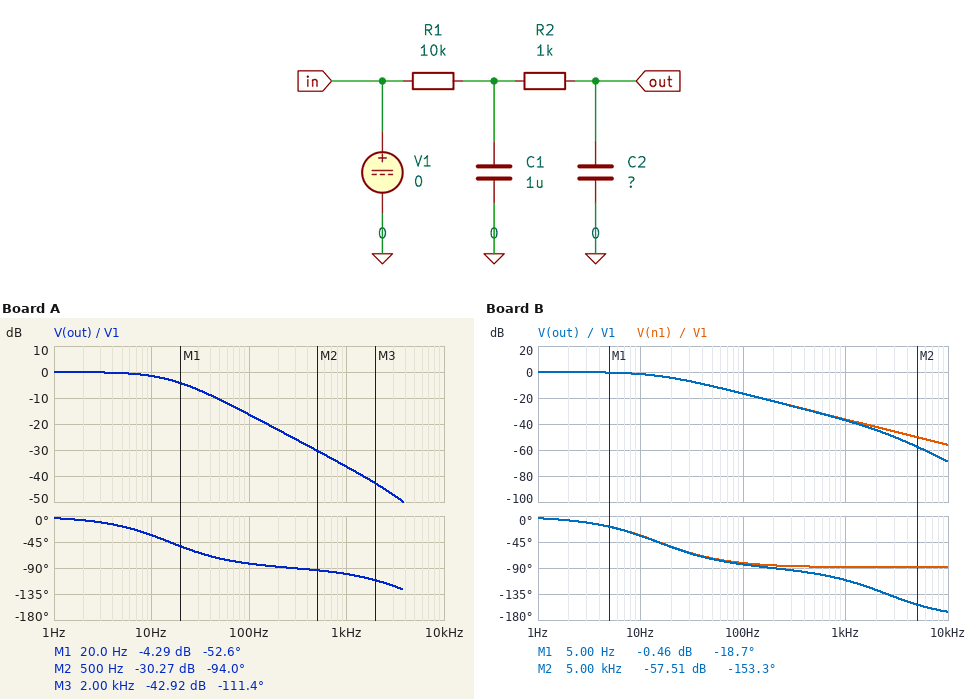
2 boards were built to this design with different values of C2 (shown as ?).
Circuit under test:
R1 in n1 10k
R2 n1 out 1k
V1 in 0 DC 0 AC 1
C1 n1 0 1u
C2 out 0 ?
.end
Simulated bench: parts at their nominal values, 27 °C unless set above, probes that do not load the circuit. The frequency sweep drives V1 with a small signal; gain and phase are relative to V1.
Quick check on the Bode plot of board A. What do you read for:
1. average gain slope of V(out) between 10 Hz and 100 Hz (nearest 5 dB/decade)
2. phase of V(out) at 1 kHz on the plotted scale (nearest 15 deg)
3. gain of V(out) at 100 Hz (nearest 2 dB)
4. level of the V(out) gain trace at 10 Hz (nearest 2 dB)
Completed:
-15 dB/decade
-105 deg
-16 dB
-2 dB
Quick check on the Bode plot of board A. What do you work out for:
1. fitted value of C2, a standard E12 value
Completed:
33 nF
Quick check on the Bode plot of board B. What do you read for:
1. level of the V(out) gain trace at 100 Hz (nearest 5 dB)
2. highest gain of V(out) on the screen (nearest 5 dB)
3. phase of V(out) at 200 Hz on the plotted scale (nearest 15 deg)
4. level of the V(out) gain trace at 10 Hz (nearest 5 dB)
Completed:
-15 dB
0 dB
-90 deg
0 dB
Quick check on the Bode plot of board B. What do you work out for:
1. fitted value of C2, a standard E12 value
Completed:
68 nF
